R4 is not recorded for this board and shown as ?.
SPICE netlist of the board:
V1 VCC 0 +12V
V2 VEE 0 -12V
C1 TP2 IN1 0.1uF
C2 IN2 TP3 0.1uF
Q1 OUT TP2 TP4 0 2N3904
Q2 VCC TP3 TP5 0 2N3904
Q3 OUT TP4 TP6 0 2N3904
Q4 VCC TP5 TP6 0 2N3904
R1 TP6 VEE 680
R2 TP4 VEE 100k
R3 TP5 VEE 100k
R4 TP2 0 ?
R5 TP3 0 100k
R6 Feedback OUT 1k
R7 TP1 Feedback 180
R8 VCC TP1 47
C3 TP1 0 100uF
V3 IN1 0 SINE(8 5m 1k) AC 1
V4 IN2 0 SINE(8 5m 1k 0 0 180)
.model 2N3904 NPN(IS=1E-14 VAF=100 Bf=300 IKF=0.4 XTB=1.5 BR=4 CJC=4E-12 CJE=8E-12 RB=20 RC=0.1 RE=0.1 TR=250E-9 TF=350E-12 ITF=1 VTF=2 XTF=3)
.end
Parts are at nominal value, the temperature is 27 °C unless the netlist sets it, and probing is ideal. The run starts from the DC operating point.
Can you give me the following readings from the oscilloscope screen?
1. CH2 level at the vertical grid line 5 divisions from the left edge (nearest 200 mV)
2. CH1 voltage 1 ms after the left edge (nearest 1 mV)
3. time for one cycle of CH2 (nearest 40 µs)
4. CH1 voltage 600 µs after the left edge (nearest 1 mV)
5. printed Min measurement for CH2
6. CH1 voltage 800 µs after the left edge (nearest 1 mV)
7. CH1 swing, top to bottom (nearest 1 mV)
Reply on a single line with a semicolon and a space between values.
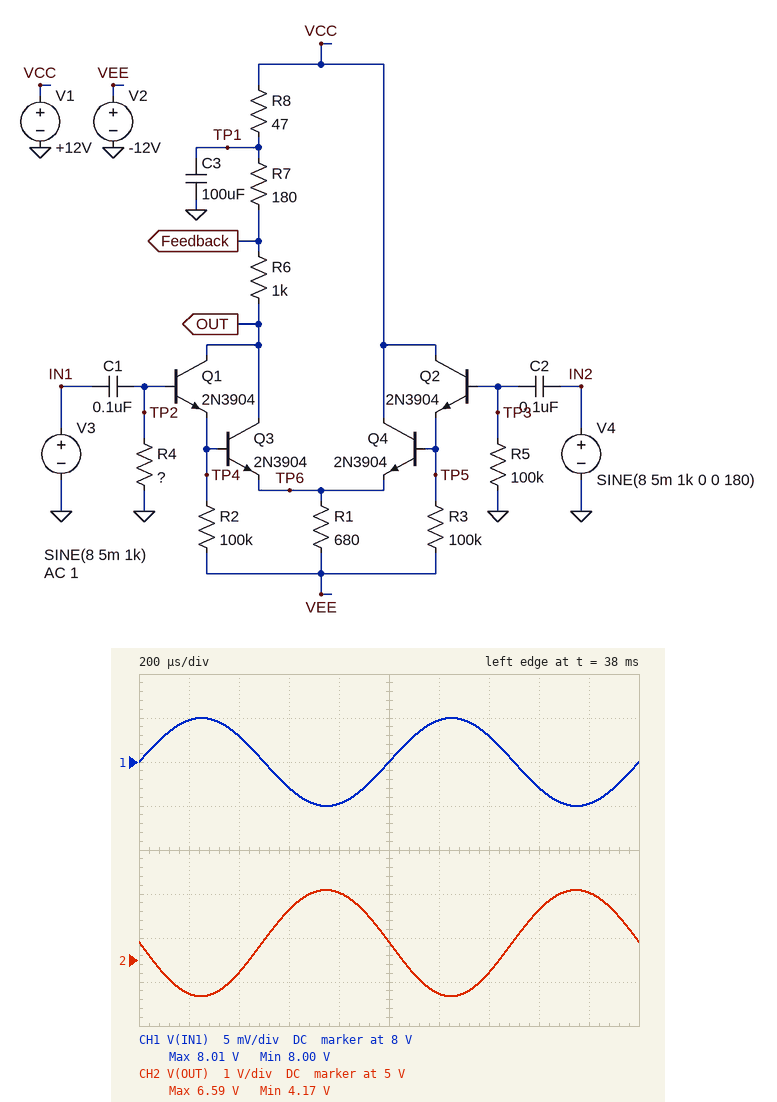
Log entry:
5.4 V; 8.000 V; 1.00 ms; 7.997 V; 4.17 V; 7.995 V; 10 mV
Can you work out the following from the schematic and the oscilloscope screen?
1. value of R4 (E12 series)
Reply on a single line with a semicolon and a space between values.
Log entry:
150 kΩ
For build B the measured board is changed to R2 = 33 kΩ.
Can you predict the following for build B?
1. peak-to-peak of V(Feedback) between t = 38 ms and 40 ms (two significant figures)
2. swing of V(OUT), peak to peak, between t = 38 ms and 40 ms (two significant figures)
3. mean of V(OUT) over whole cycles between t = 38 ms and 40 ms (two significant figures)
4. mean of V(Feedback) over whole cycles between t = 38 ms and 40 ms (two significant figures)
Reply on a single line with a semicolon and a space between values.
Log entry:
20 mV; 130 mV; 11 V; 12 V
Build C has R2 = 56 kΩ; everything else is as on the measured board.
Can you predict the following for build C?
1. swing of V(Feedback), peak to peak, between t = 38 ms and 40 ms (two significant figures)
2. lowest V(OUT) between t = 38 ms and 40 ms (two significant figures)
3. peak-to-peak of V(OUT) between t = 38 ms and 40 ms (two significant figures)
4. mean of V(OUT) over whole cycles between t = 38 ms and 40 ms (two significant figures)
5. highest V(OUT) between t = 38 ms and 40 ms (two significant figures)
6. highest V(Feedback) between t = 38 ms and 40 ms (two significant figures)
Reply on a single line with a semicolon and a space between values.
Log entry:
190 mV; 8.9 V; 1.3 V; 9.6 V; 10 V; 12 V
